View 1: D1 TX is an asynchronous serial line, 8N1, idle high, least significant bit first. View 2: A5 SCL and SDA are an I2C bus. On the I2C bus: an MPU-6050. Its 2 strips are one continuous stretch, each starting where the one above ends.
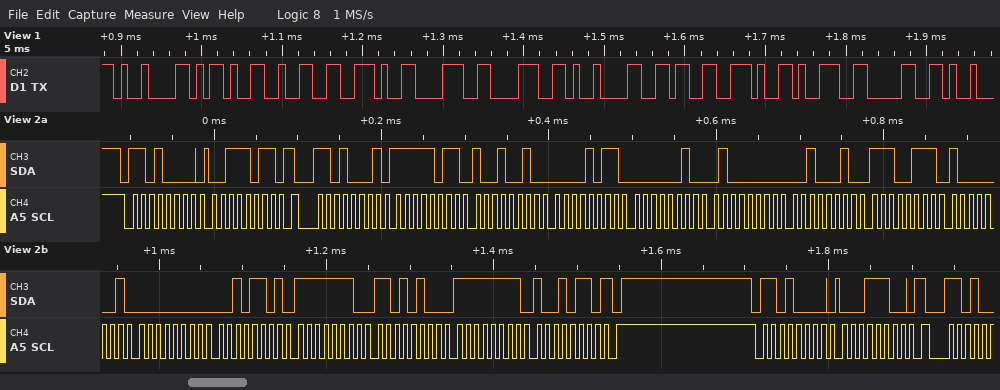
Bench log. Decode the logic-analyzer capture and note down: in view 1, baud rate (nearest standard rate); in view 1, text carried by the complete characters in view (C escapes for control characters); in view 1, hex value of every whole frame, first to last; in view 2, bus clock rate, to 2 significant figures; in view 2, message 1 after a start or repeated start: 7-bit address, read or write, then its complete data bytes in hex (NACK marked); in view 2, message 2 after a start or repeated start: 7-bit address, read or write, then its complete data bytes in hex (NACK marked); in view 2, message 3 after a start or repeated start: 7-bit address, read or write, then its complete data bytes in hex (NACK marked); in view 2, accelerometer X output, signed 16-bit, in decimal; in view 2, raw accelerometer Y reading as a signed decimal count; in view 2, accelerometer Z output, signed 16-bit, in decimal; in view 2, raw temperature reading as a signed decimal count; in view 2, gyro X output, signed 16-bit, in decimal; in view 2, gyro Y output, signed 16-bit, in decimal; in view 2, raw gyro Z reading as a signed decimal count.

115200 baud
"\t-2.88\t6.90"
09 2D 32 2E 38 38 09 36 2E 39 30
100 kHz
0x68 write: 3B
0x68 read: FB 92 0B 02 40 22 E7 81 00 2D FE D4 FF 96 NACK
0x68 write: 1C
-1134
2818
16418
-6271
45
-300
-106
